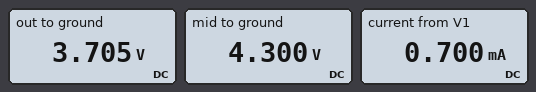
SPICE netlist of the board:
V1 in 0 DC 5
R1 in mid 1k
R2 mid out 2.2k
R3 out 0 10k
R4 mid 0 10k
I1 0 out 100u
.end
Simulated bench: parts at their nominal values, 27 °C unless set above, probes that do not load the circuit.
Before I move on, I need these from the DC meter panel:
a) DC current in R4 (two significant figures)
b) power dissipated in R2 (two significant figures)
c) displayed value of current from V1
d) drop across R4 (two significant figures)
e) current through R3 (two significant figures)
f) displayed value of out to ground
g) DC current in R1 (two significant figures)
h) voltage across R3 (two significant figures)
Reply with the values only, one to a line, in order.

430 µA
160 µW
0.700 mA
4.3 V
370 µA
3.705 V
700 µA
3.7 V
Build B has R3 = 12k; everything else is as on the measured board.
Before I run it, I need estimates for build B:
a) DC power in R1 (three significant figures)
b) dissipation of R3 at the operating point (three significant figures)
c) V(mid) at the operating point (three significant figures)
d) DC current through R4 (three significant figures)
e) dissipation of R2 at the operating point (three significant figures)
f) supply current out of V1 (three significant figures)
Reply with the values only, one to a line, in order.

430 µW
1.24 mW
4.34 V
434 µA
108 µW
656 µA
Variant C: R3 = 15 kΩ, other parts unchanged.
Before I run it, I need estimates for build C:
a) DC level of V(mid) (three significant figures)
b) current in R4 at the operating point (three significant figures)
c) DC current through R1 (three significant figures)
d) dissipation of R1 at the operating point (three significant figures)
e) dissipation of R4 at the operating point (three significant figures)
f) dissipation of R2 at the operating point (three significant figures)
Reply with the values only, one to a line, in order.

4.39 V
439 µA
607 µA
369 µW
1.93 mW
62.2 µW
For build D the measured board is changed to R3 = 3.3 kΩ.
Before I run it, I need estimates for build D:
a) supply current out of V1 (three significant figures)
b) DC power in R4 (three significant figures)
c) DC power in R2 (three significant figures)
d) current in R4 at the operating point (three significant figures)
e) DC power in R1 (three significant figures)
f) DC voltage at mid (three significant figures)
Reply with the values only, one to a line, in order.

1.05 mA
1.56 mW
952 µW
395 µA
1.11 mW
3.95 V
